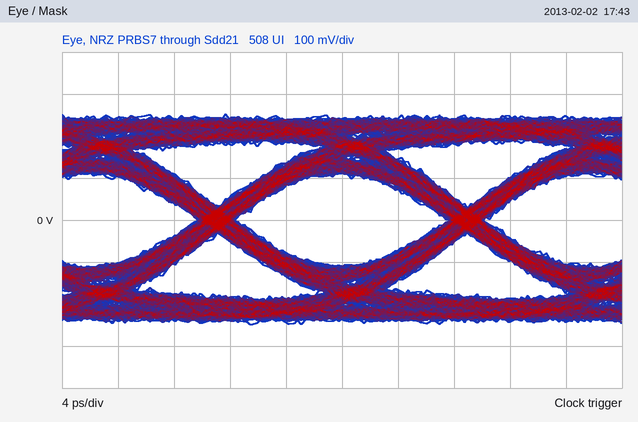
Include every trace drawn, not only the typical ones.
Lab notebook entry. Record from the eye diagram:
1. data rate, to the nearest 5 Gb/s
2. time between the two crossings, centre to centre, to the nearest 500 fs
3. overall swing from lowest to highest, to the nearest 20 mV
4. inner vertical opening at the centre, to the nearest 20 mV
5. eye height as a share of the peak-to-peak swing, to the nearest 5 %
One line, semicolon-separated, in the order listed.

55 Gb/s; 18.0 ps; 500 mV; 220 mV; 45 %
